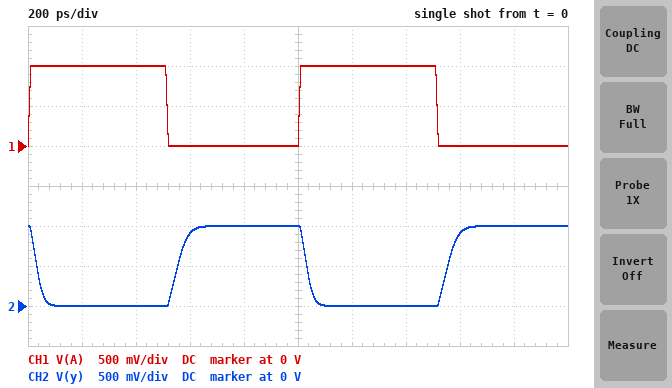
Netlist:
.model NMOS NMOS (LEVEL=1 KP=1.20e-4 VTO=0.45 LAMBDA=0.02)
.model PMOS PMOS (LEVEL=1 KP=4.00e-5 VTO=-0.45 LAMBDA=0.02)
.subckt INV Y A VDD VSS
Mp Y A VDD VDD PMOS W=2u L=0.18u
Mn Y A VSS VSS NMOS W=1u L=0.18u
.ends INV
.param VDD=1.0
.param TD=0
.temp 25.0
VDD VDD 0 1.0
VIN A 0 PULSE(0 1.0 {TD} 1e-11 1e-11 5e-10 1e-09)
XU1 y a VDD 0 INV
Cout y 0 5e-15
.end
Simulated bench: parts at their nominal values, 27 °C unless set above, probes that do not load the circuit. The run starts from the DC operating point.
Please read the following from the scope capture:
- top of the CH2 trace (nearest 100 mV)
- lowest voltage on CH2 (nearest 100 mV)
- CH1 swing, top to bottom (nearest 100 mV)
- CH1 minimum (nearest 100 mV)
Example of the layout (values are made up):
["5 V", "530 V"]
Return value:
["1.0 V", "0 V", "1.0 V", "0 V"]
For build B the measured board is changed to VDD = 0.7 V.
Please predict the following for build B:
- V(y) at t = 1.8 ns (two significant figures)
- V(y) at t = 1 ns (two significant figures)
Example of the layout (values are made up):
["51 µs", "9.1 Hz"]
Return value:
["670 mV", "700 mV"]
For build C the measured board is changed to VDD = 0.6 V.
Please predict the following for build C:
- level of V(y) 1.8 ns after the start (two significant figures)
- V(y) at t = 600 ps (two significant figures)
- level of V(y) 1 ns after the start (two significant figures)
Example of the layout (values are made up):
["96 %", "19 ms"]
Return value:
["280 mV", "80 mV", "470 mV"]
